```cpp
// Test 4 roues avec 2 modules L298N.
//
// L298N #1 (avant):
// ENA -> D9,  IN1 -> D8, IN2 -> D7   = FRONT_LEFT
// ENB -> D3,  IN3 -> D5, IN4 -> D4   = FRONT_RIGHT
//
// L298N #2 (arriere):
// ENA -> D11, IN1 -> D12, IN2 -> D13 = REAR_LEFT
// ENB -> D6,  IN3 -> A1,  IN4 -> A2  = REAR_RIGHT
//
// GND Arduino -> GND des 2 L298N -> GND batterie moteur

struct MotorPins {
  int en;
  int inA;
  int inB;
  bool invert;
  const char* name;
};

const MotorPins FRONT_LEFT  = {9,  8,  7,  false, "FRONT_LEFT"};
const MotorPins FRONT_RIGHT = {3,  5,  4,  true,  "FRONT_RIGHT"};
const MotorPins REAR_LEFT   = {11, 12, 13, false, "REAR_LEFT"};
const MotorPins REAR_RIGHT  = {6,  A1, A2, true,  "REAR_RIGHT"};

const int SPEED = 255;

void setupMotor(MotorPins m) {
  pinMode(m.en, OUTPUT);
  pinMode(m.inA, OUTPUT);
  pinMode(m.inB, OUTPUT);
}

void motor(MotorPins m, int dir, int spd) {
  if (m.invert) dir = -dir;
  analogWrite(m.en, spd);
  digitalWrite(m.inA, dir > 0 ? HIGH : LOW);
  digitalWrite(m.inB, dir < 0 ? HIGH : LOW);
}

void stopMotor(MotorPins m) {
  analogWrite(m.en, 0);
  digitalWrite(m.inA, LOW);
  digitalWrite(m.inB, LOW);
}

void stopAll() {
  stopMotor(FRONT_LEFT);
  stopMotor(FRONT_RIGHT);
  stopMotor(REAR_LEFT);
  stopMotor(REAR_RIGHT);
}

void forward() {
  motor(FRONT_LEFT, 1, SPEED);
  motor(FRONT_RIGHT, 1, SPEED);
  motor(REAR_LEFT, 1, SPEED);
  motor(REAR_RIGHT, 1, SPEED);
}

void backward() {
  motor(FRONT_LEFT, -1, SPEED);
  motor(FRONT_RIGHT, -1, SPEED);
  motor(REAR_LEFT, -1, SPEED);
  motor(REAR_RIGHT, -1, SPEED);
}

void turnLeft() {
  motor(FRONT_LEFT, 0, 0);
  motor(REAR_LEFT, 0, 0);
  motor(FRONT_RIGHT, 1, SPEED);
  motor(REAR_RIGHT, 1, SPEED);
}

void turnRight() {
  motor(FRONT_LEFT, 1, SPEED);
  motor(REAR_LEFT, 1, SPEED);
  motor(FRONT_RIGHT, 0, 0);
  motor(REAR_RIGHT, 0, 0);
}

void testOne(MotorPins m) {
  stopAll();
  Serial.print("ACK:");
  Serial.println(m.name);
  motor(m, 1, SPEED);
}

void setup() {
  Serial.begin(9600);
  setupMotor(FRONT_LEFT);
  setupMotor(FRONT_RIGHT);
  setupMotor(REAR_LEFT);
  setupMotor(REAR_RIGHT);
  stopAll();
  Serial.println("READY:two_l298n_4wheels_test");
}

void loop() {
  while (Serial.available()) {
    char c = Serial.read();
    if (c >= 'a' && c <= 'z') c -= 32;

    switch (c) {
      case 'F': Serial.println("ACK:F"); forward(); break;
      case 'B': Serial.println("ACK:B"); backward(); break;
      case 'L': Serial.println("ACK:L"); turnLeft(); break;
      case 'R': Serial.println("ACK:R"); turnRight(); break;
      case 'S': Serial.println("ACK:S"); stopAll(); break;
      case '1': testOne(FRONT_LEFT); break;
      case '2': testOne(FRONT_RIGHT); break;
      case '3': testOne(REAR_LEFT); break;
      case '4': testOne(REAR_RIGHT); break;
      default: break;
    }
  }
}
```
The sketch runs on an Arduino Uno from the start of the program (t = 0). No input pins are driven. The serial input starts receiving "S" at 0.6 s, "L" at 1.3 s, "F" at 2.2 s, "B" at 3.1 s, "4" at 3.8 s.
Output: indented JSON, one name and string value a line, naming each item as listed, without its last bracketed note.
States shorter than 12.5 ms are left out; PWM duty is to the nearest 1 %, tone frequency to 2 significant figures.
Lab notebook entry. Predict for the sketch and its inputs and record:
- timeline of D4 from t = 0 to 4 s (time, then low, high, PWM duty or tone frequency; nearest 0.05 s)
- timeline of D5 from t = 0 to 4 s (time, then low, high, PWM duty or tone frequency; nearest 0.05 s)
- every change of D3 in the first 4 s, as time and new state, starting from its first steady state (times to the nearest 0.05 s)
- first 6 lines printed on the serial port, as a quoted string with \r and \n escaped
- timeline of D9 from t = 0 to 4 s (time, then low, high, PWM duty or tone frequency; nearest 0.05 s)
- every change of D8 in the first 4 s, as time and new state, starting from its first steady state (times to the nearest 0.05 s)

{
  "timeline of D4 from t = 0 to 4 s": "0 s low; 1.3 s high; 3.1 s low",
  "timeline of D5 from t = 0 to 4 s": "0 s low; 3.1 s high; 3.8 s low",
  "every change of D3 in the first 4 s, as time and new state, starting from its first steady state": "0 s low; 1.3 s high; 3.8 s low",
  "first 6 lines printed on the serial port, as a quoted string with \\r and \\n escaped": "\"READY:two_l298n_4wheels_test\\r\\nACK:S\\r\\nACK:L\\r\\nACK:F\\r\\nACK:B\\r\\nACK:REAR_RIGHT\\r\\n\"",
  "timeline of D9 from t = 0 to 4 s": "0 s low; 2.2 s high; 3.8 s low",
  "every change of D8 in the first 4 s, as time and new state, starting from its first steady state": "0 s low; 2.2 s high; 3.1 s low"
}
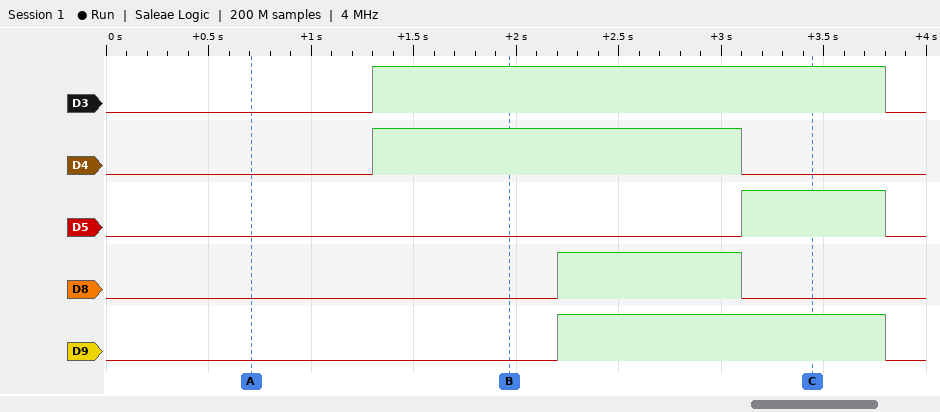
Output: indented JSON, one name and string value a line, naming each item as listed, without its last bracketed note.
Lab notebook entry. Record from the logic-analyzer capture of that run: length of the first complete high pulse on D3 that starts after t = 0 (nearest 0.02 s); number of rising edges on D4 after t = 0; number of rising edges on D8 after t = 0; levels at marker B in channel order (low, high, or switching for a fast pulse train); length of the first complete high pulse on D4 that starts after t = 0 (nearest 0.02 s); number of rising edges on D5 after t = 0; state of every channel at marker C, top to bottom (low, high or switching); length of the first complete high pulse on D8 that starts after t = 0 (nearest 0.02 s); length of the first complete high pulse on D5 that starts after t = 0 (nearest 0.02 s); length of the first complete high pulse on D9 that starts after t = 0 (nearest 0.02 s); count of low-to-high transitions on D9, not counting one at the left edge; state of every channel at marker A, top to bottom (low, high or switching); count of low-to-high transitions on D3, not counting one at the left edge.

{
  "length of the first complete high pulse on D3 that starts after t = 0": "2.50 s",
  "number of rising edges on D4 after t = 0": "1",
  "number of rising edges on D8 after t = 0": "1",
  "levels at marker B in channel order": "D3 high, D4 high, D5 low, D8 low, D9 low",
  "length of the first complete high pulse on D4 that starts after t = 0": "1.80 s",
  "number of rising edges on D5 after t = 0": "1",
  "state of every channel at marker C, top to bottom": "D3 high, D4 low, D5 high, D8 low, D9 high",
  "length of the first complete high pulse on D8 that starts after t = 0": "0.90 s",
  "length of the first complete high pulse on D5 that starts after t = 0": "0.70 s",
  "length of the first complete high pulse on D9 that starts after t = 0": "1.60 s",
  "count of low-to-high transitions on D9, not counting one at the left edge": "1",
  "state of every channel at marker A, top to bottom": "D3 low, D4 low, D5 low, D8 low, D9 low",
  "count of low-to-high transitions on D3, not counting one at the left edge": "1"
}
